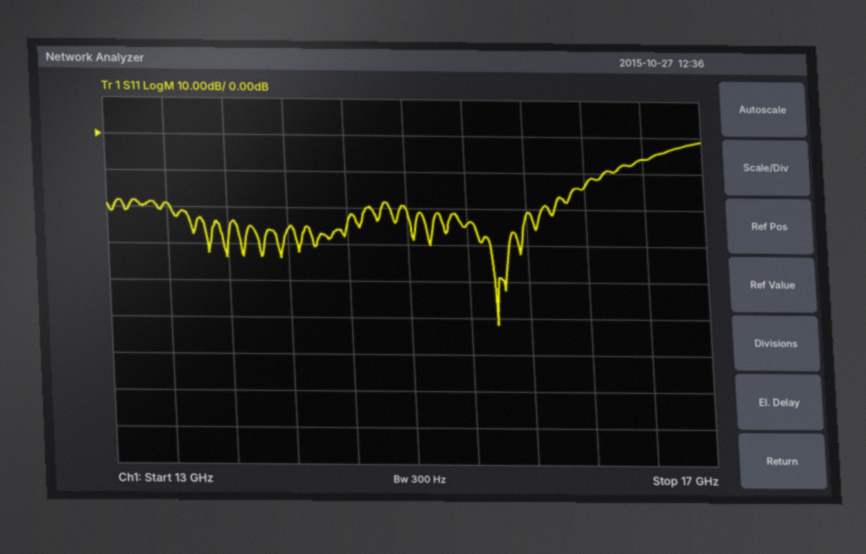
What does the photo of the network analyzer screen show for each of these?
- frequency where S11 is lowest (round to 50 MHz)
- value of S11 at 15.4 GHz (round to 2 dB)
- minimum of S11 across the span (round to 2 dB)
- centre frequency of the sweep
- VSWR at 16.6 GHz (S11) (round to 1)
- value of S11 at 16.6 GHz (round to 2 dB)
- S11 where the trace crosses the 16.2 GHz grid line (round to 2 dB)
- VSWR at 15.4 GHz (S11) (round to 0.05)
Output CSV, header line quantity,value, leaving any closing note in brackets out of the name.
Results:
quantity,value
frequency where S11 is lowest,15.60 GHz
value of S11 at 15.4 GHz,-24 dB
minimum of S11 across the span,-52 dB
centre frequency of the sweep,15 GHz
VSWR at 16.6 GHz (S11),3
value of S11 at 16.6 GHz,-6 dB
S11 where the trace crosses the 16.2 GHz grid line,-14 dB
VSWR at 15.4 GHz (S11),1.15
